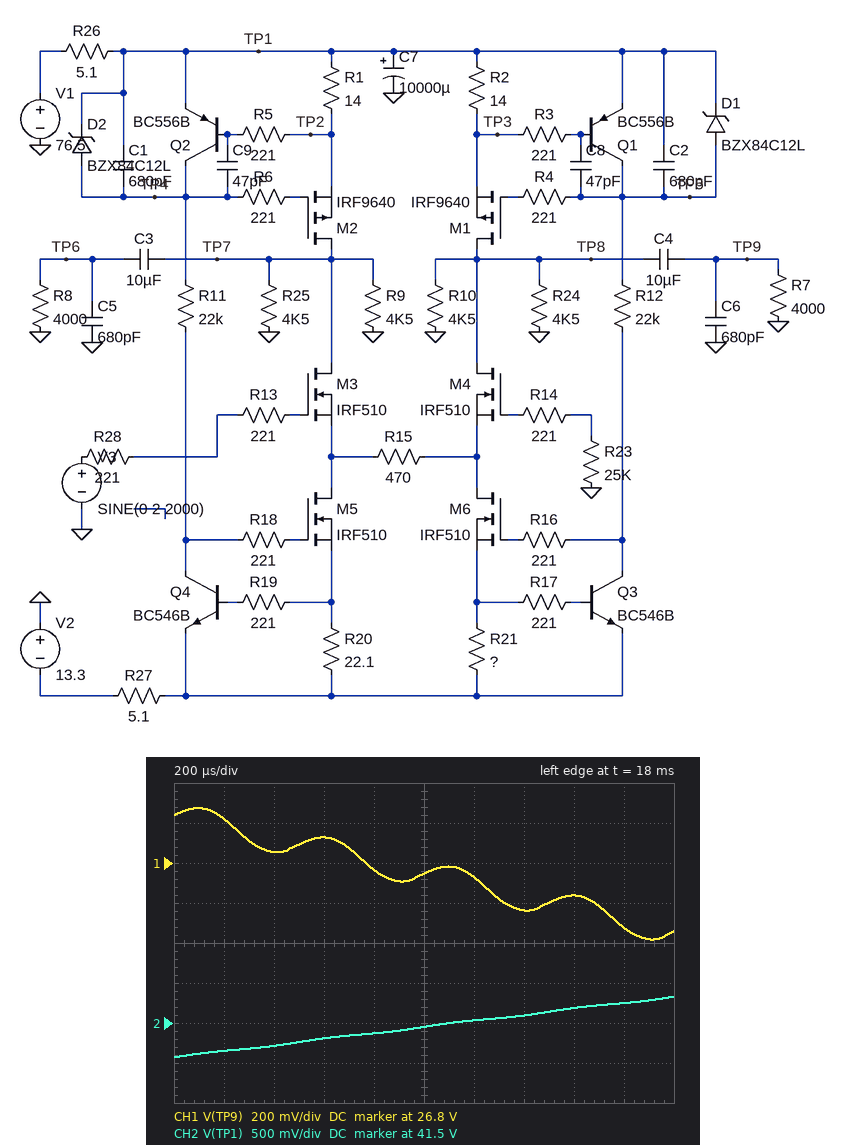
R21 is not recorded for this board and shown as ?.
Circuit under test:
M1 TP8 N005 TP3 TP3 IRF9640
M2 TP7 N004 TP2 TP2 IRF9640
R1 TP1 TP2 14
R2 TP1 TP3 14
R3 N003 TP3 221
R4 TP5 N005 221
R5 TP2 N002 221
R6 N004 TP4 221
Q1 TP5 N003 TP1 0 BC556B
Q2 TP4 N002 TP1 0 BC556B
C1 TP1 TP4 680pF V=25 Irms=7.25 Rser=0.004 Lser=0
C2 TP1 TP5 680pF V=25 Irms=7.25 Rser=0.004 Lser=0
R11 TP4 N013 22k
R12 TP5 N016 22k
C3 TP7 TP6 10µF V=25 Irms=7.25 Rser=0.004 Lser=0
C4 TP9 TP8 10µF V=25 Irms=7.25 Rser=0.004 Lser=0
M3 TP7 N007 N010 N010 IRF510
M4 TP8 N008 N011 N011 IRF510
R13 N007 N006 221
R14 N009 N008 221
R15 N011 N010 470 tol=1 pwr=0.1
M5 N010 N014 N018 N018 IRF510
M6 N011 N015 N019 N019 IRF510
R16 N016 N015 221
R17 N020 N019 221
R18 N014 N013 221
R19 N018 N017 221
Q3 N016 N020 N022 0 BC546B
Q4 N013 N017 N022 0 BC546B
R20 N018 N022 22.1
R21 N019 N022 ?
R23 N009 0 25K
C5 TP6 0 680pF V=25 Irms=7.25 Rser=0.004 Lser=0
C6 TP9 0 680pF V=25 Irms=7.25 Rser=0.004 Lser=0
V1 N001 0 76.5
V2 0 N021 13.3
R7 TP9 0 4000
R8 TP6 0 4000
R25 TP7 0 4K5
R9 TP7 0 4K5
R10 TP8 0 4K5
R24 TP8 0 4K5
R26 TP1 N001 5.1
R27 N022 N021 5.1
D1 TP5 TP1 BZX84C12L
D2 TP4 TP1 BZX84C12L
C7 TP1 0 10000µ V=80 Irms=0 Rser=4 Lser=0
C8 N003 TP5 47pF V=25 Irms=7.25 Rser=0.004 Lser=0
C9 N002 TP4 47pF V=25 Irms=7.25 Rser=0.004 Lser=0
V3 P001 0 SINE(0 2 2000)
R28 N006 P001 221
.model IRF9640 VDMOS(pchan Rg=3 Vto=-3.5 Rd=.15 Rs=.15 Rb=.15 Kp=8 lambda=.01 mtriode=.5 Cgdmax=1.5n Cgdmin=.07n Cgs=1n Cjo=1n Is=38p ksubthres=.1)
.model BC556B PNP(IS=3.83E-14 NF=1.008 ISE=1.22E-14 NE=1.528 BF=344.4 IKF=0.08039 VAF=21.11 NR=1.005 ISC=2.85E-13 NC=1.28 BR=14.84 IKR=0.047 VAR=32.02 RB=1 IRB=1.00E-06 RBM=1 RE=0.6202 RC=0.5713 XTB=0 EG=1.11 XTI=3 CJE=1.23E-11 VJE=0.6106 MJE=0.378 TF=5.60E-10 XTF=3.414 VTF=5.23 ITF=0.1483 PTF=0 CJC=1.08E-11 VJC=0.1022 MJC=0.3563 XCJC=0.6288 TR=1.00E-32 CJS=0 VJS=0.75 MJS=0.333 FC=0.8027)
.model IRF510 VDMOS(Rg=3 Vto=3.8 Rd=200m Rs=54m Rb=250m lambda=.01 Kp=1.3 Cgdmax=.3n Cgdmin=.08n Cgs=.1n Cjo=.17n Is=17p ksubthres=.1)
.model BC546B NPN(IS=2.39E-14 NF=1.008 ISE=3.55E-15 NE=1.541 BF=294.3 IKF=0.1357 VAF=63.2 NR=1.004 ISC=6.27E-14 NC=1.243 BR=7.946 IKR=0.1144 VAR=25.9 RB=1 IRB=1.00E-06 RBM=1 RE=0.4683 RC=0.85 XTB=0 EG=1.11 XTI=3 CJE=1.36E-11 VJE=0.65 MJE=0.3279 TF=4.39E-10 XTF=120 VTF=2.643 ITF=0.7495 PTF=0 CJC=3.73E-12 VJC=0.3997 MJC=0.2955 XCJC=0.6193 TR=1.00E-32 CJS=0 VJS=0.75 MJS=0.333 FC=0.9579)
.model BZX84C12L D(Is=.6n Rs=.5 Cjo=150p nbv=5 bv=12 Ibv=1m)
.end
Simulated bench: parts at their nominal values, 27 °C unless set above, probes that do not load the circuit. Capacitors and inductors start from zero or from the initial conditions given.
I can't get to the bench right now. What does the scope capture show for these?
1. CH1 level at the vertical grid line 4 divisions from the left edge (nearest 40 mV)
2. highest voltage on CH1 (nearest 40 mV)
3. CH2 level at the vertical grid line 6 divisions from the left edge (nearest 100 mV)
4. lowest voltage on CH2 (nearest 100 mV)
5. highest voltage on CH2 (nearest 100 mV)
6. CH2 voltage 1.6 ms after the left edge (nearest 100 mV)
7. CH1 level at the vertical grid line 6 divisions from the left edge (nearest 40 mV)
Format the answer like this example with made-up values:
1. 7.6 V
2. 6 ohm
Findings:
1. 26.76 V
2. 27.08 V
3. 41.5 V
4. 41.1 V
5. 41.8 V
6. 41.7 V
7. 26.72 V
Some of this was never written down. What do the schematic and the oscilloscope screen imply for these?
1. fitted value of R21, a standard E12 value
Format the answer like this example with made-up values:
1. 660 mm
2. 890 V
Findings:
1. 39 Ω
